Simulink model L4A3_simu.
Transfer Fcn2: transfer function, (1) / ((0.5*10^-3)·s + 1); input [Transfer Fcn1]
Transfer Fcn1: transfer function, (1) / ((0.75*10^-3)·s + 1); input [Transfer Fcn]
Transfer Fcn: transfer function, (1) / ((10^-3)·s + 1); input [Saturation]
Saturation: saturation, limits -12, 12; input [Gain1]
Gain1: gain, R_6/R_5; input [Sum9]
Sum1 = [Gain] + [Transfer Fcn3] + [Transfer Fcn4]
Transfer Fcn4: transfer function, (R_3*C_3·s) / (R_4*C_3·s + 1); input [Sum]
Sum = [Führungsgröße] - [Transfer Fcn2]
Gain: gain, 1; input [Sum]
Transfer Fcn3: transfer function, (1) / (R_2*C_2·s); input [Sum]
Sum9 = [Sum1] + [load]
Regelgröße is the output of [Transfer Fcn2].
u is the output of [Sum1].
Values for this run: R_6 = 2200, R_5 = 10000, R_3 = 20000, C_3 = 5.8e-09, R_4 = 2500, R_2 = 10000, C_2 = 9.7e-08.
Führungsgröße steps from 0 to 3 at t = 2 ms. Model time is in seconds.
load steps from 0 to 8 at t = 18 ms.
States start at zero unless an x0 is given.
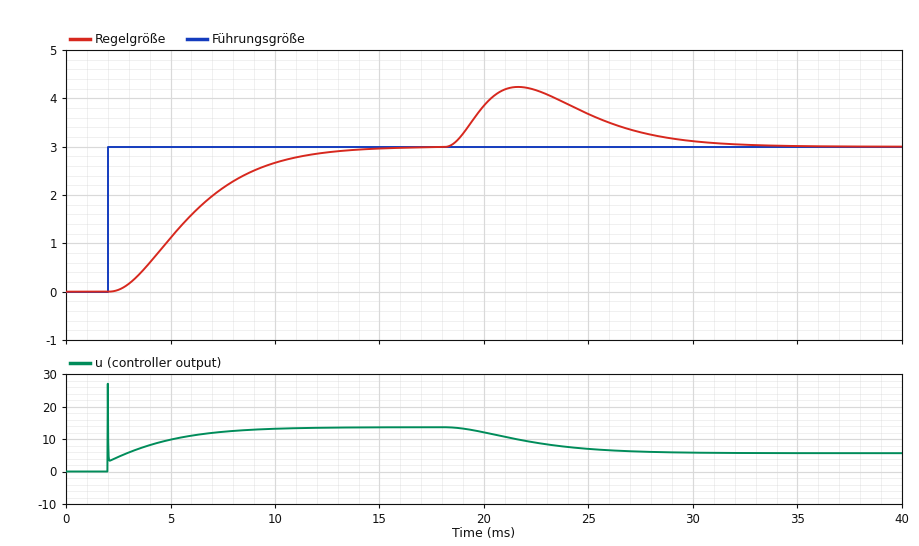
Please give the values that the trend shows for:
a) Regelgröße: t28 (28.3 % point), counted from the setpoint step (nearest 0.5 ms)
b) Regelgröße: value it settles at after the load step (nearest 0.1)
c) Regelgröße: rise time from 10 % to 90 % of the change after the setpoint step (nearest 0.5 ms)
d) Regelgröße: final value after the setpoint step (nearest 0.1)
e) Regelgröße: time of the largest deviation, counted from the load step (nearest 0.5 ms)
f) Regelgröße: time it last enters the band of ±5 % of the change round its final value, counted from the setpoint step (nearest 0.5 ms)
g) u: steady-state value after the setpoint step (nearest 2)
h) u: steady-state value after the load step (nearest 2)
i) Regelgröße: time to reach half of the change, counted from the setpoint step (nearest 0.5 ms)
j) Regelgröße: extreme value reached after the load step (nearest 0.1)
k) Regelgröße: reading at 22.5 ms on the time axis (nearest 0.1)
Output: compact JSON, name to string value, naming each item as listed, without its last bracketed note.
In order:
{"Regelgröße: t28 (28.3 % point), counted from the setpoint step": "2.5 ms", "Regelgröße: value it settles at after the load step": "3.0", "Regelgröße: rise time from 10 % to 90 % of the change after the setpoint step": "7.0 ms", "Regelgröße: final value after the setpoint step": "3.0", "Regelgröße: time of the largest deviation, counted from the load step": "3.5 ms", "Regelgröße: time it last enters the band of ±5 % of the change round its final value, counted from the setpoint step": "10.0 ms", "u: steady-state value after the setpoint step": "14", "u: steady-state value after the load step": "6", "Regelgröße: time to reach half of the change, counted from the setpoint step": "4.0 ms", "Regelgröße: extreme value reached after the load step": "4.2", "Regelgröße: reading at 22.5 ms on the time axis": "4.2"}
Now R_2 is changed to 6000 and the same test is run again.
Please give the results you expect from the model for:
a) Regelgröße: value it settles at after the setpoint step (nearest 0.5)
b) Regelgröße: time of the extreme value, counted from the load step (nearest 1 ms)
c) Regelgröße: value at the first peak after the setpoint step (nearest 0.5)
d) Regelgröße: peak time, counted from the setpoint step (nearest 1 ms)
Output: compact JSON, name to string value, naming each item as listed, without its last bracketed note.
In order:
{"Regelgröße: value it settles at after the setpoint step": "3.0", "Regelgröße: time of the extreme value, counted from the load step": "3 ms", "Regelgröße: value at the first peak after the setpoint step": "3.5", "Regelgröße: peak time, counted from the setpoint step": "8 ms"}
